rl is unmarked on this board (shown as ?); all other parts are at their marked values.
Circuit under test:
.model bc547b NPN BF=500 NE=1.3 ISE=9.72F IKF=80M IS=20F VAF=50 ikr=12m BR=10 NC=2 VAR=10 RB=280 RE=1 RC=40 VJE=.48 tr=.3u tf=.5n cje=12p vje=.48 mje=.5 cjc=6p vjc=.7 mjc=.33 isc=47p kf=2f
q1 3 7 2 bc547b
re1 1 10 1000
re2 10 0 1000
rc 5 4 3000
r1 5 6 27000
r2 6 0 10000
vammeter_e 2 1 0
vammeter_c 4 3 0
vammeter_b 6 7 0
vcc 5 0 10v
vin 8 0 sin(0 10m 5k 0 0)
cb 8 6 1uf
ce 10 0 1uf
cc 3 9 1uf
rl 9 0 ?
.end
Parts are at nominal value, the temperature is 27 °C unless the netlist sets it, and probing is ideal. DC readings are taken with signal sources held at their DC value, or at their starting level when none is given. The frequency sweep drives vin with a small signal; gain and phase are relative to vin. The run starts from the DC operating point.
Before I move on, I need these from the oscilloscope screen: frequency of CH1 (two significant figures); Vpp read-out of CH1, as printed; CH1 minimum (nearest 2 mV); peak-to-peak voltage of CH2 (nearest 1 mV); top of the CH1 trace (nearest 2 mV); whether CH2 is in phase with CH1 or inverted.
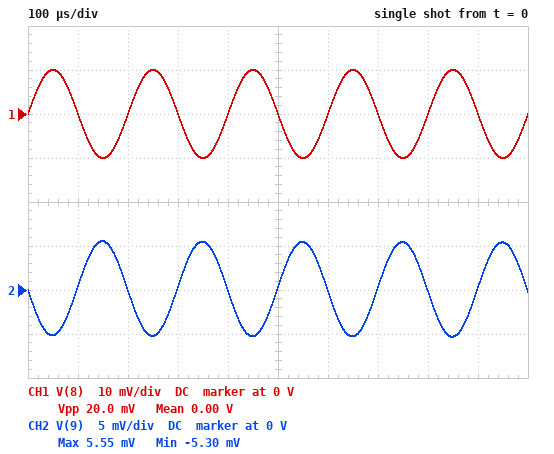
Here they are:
5.0 kHz
20.0 mV
-10 mV
11 mV
10 mV
inverted
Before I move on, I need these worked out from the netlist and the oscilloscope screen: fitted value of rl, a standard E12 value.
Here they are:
680 Ω
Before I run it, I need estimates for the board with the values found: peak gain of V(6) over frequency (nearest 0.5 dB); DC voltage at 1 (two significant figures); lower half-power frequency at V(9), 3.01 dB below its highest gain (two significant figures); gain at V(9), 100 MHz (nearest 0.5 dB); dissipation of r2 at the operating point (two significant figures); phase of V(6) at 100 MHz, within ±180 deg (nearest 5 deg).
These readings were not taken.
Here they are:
0 dB
2.0 V
280 Hz
-5.0 dB
720 µW
0 deg
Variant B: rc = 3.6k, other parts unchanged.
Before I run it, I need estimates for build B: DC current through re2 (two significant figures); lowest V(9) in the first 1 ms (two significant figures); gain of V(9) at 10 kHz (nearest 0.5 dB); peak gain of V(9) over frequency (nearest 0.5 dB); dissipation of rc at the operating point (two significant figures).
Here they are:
1.0 mA
-5.5 mV
-5.0 dB
-4.5 dB
3.7 mW
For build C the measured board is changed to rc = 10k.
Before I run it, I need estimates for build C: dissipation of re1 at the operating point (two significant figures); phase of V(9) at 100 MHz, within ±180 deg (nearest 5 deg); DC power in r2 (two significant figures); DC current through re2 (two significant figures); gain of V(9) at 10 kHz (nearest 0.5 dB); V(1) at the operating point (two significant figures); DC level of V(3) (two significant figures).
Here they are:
750 µW
0 deg
570 µW
860 µA
-15.5 dB
1.7 V
1.8 V
